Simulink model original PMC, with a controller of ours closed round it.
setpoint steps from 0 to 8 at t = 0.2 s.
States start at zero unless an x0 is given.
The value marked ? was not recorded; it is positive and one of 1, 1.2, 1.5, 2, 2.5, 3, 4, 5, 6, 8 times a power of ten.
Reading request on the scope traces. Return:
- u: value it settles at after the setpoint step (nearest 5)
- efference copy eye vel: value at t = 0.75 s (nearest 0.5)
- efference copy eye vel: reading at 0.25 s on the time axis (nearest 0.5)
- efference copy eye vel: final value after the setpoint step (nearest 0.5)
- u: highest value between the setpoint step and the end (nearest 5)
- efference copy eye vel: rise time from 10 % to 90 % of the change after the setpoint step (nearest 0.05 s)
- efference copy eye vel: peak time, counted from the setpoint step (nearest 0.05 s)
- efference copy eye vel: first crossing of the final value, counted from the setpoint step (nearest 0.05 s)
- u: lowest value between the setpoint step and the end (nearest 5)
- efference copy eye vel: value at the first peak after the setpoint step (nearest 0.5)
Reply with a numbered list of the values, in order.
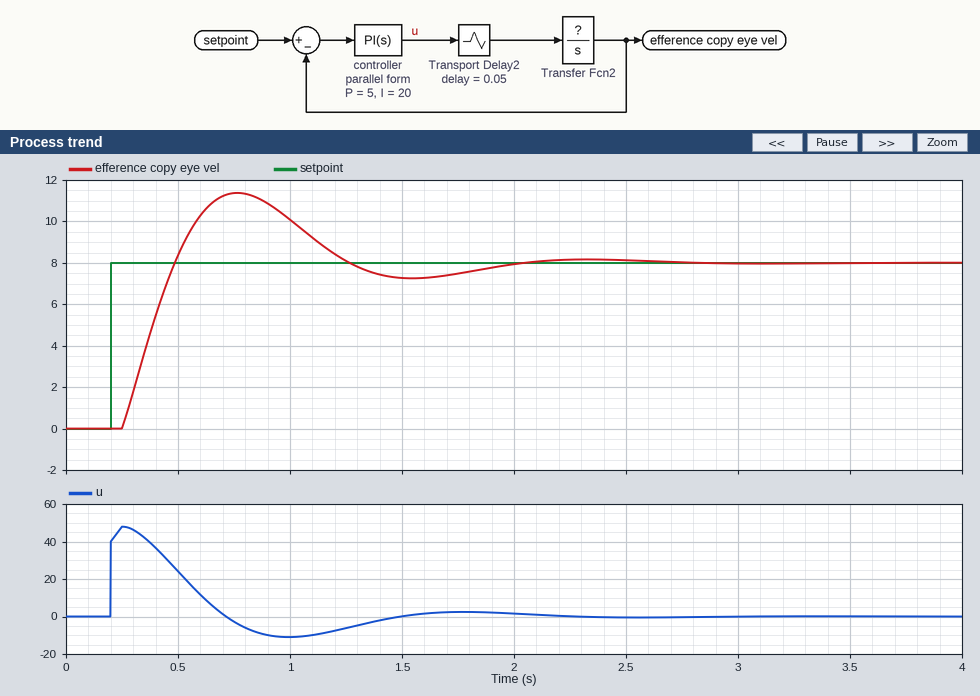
1. 0
2. 11.5
3. 0.0
4. 8.0
5. 50
6. 0.20 s
7. 0.55 s
8. 0.30 s
9. -10
10. 11.5
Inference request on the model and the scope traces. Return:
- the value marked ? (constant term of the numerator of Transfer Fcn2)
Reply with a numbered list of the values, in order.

1. 0.8
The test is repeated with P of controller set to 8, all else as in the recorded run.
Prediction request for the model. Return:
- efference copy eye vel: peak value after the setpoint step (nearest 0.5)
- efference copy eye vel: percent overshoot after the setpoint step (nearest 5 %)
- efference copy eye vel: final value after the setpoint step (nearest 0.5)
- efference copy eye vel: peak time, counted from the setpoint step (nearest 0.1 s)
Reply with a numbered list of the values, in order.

1. 10.0
2. 25 %
3. 8.0
4. 0.4 s
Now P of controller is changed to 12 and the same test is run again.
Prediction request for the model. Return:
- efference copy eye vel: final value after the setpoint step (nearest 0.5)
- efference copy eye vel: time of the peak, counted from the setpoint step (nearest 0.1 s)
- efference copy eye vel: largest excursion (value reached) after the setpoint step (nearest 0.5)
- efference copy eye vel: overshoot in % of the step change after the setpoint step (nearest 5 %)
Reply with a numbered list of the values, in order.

1. 8.0
2. 0.3 s
3. 9.5
4. 20 %
